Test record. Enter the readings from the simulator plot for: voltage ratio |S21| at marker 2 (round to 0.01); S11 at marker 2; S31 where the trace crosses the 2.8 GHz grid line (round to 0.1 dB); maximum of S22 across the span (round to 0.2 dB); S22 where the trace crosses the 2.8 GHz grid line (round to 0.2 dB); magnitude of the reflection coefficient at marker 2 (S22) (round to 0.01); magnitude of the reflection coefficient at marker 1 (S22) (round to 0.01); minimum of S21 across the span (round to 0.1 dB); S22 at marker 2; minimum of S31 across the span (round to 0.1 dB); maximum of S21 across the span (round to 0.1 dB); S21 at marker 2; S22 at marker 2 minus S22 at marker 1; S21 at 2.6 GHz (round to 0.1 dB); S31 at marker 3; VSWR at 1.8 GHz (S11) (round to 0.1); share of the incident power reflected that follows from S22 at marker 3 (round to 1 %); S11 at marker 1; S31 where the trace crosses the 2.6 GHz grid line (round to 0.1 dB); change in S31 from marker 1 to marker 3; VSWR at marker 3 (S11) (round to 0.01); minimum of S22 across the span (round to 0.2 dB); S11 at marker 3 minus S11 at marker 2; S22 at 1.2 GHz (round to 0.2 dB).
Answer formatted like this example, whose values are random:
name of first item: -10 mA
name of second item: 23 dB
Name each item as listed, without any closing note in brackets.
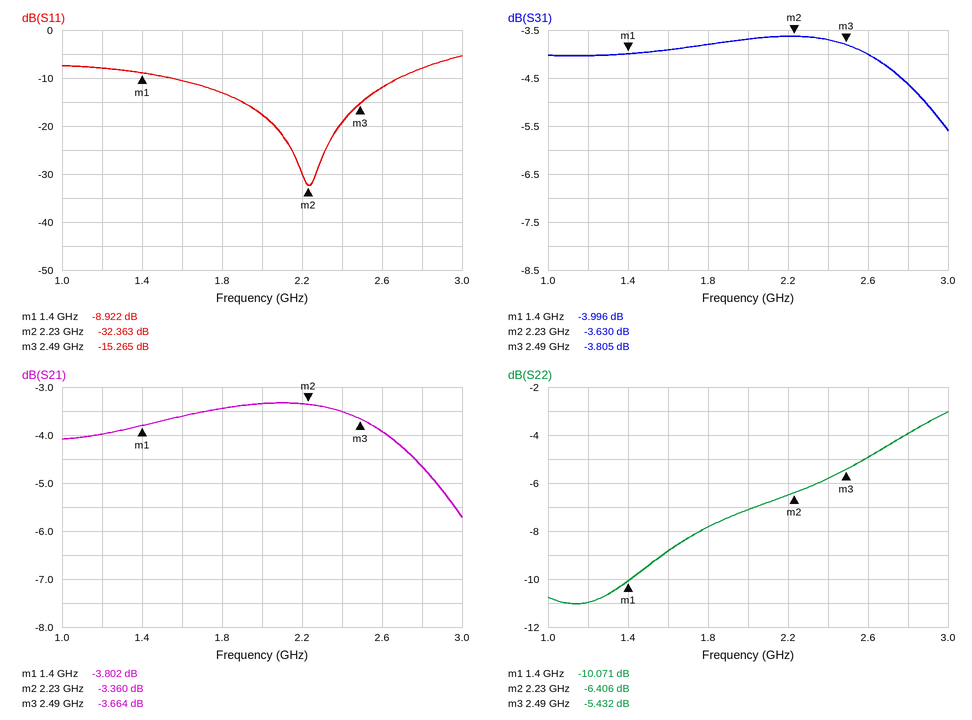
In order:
voltage ratio |S21| at marker 2: 0.68
S11 at marker 2: -32.363 dB
S31 where the trace crosses the 2.8 GHz grid line: -4.6 dB
maximum of S22 across the span: -3.0 dB
S22 where the trace crosses the 2.8 GHz grid line: -4.0 dB
magnitude of the reflection coefficient at marker 2 (S22): 0.48
magnitude of the reflection coefficient at marker 1 (S22): 0.31
minimum of S21 across the span: -5.7 dB
S22 at marker 2: -6.406 dB
minimum of S31 across the span: -5.6 dB
maximum of S21 across the span: -3.3 dB
S21 at marker 2: -3.360 dB
S22 at marker 2 minus S22 at marker 1: 3.665 dB
S21 at 2.6 GHz: -3.9 dB
S31 at marker 3: -3.805 dB
VSWR at 1.8 GHz (S11): 1.6
share of the incident power reflected that follows from S22 at marker 3: 29 %
S11 at marker 1: -8.922 dB
S31 where the trace crosses the 2.6 GHz grid line: -4.0 dB
change in S31 from marker 1 to marker 3: 0.191 dB
VSWR at marker 3 (S11): 1.42
minimum of S22 across the span: -11.0 dB
S11 at marker 3 minus S11 at marker 2: 17.098 dB
S22 at 1.2 GHz: -11.0 dB
